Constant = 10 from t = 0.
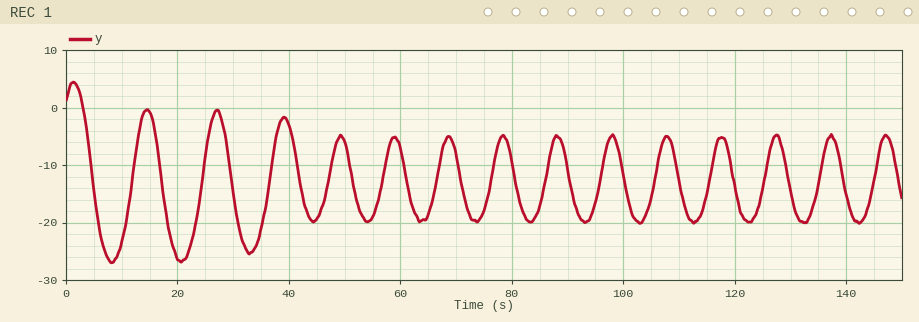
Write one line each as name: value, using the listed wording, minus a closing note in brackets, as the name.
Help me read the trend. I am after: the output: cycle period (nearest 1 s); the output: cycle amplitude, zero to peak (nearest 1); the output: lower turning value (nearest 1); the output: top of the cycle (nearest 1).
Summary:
the output: cycle period: 10 s
the output: cycle amplitude, zero to peak: 8
the output: lower turning value: -20
the output: top of the cycle: -5
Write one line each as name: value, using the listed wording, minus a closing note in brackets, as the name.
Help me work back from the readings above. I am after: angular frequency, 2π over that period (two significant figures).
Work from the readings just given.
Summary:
angular frequency, 2π over that period: 0.63 rad/s
